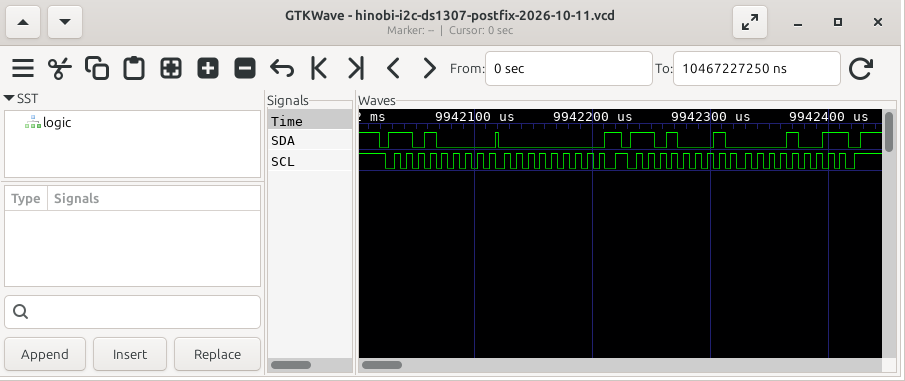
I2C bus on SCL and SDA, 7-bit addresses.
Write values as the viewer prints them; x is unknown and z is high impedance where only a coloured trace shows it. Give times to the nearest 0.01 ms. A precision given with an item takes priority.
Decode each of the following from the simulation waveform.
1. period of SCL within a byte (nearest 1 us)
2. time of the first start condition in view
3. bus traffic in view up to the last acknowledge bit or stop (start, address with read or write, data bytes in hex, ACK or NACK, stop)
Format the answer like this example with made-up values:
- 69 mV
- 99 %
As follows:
- 10 us
- 9942.02 ms
- start, address 68 write ACK, 00 ACK, repeated start, address 68 read ACK, 09 NACK, stop
